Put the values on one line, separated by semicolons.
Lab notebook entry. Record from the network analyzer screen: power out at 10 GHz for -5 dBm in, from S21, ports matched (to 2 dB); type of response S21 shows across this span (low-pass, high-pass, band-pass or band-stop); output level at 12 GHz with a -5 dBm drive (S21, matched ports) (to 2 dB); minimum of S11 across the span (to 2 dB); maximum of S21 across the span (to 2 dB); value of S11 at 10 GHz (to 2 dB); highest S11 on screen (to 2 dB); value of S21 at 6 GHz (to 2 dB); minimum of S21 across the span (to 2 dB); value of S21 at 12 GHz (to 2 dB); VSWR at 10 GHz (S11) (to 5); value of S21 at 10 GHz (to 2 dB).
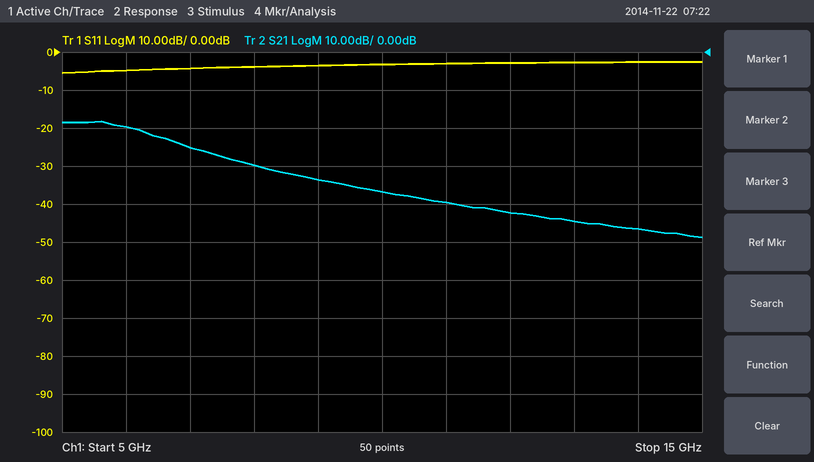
-42 dBm; low-pass; -48 dBm; -6 dB; -18 dB; -4 dB; -2 dB; -20 dB; -48 dB; -42 dB; 5; -36 dB
